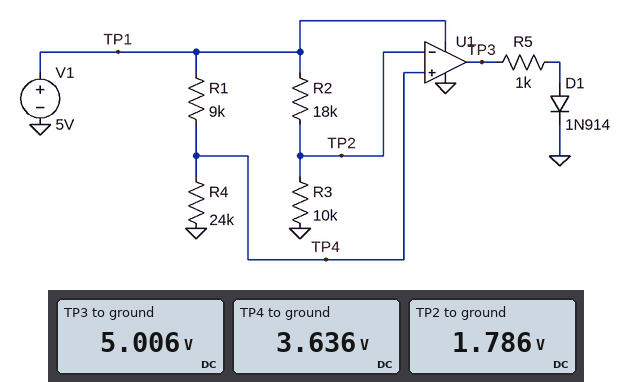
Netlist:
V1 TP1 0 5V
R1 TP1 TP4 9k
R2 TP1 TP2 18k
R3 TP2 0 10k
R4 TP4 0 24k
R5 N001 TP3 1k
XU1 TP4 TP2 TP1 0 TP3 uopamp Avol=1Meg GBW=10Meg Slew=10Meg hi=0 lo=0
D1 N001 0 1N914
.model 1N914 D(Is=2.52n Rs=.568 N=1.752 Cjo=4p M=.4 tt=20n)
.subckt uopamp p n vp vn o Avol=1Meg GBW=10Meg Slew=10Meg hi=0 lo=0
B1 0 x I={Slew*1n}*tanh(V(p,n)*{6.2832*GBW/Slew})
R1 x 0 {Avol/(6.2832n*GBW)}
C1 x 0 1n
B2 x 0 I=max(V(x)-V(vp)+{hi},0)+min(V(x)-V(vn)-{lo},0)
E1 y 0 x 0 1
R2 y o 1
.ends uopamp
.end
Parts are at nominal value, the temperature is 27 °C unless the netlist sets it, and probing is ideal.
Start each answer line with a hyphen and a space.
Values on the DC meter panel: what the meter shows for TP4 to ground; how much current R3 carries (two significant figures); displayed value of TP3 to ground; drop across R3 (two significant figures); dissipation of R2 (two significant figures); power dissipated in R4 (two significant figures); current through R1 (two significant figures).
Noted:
- 3.636 V
- 180 µA
- 5.006 V
- 1.8 V
- 570 µW
- 550 µW
- 150 µA
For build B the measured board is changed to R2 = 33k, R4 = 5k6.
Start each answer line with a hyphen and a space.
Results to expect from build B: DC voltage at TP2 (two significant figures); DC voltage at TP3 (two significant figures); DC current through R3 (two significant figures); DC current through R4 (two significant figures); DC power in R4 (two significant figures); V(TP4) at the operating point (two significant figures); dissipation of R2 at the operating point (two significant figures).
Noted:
- 1.2 V
- 5.0 V
- 120 µA
- 340 µA
- 660 µW
- 1.9 V
- 450 µW
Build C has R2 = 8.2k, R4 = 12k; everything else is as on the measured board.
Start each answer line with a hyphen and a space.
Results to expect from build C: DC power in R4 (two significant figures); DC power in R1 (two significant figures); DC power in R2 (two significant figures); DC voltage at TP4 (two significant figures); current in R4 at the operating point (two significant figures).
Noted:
- 680 µW
- 510 µW
- 620 µW
- 2.9 V
- 240 µA
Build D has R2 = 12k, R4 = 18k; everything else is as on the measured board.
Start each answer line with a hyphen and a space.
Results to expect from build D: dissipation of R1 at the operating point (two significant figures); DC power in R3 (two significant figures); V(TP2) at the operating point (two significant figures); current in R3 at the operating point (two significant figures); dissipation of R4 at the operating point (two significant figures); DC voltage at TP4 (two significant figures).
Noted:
- 310 µW
- 520 µW
- 2.3 V
- 230 µA
- 620 µW
- 3.3 V
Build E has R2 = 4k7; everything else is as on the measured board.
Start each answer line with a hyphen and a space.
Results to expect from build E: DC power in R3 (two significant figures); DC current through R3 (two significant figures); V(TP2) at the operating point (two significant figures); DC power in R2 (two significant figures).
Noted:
- 1.2 mW
- 340 µA
- 3.4 V
- 540 µW
